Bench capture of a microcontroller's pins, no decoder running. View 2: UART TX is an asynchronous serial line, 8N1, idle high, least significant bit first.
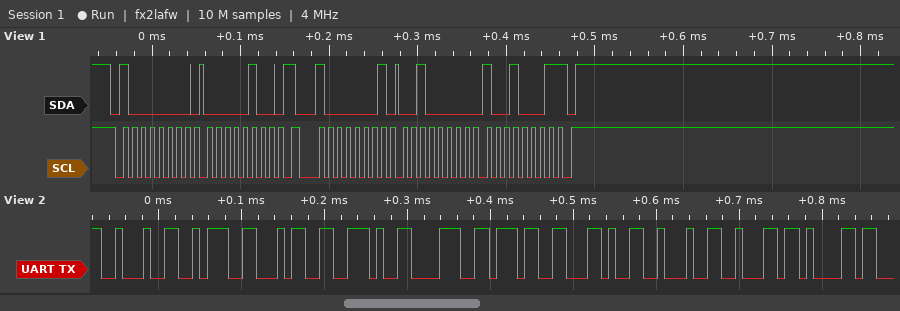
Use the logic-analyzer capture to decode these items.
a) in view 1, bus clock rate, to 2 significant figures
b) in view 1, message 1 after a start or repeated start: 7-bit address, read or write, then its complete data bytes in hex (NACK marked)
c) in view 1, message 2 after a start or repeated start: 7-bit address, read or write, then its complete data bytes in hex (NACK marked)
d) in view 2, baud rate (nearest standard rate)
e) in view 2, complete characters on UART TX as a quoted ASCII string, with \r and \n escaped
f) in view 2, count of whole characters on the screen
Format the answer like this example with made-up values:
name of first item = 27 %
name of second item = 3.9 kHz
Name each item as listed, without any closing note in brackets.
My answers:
in view 1, bus clock rate, to 2 significant figures = 100 kHz
in view 1, message 1 after a start or repeated start: 7-bit address, read or write, then its complete data bytes in hex = 0x40 write: 04
in view 1, message 2 after a start or repeated start: 7-bit address, read or write, then its complete data bytes in hex = 0x40 read: 20 91 NACK
in view 2, baud rate = 115200 baud
in view 2, complete characters on UART TX as a quoted ASCII string, with \r and \n escaped = "\":4.87,\"ba"
in view 2, count of whole characters on the screen = 10
